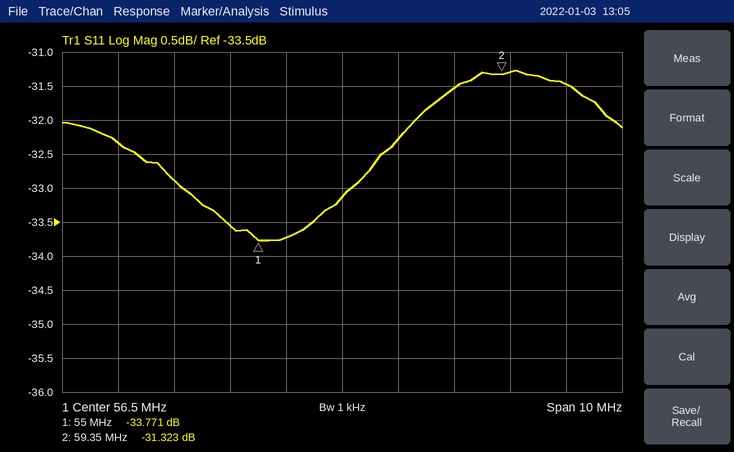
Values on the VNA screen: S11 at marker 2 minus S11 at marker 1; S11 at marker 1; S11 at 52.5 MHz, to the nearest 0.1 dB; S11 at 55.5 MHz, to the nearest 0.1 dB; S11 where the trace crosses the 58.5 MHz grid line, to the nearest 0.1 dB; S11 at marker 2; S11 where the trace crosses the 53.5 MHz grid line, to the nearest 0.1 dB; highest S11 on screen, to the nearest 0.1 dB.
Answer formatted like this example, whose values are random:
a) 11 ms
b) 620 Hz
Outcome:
a) 2.448 dB
b) -33.771 dB
c) -32.3 dB
d) -33.7 dB
e) -31.5 dB
f) -31.323 dB
g) -32.9 dB
h) -31.3 dB
